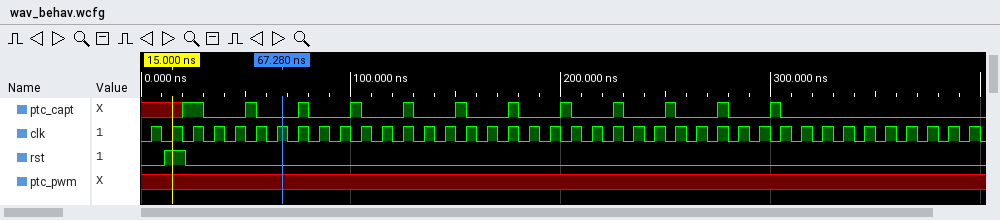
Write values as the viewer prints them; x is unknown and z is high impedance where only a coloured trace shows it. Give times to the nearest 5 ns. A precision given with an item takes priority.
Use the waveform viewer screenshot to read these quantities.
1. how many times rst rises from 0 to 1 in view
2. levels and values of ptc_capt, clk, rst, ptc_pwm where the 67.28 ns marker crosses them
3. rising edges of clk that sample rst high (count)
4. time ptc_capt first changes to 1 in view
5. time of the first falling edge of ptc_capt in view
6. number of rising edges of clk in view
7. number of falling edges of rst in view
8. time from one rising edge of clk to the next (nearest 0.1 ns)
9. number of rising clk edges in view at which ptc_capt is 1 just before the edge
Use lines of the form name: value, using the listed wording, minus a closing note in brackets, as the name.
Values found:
how many times rst rises from 0 to 1 in view: 1
levels and values of ptc_capt, clk, rst, ptc_pwm where the 67.28 ns marker crosses them: ptc_capt=0, clk=1, rst=0, ptc_pwm=x
rising edges of clk that sample rst high: 1
time ptc_capt first changes to 1 in view: 20 ns
time of the first falling edge of ptc_capt in view: 30 ns
number of rising edges of clk in view: 40
number of falling edges of rst in view: 1
time from one rising edge of clk to the next: 10 ns
number of rising clk edges in view at which ptc_capt is 1 just before the edge: 7
